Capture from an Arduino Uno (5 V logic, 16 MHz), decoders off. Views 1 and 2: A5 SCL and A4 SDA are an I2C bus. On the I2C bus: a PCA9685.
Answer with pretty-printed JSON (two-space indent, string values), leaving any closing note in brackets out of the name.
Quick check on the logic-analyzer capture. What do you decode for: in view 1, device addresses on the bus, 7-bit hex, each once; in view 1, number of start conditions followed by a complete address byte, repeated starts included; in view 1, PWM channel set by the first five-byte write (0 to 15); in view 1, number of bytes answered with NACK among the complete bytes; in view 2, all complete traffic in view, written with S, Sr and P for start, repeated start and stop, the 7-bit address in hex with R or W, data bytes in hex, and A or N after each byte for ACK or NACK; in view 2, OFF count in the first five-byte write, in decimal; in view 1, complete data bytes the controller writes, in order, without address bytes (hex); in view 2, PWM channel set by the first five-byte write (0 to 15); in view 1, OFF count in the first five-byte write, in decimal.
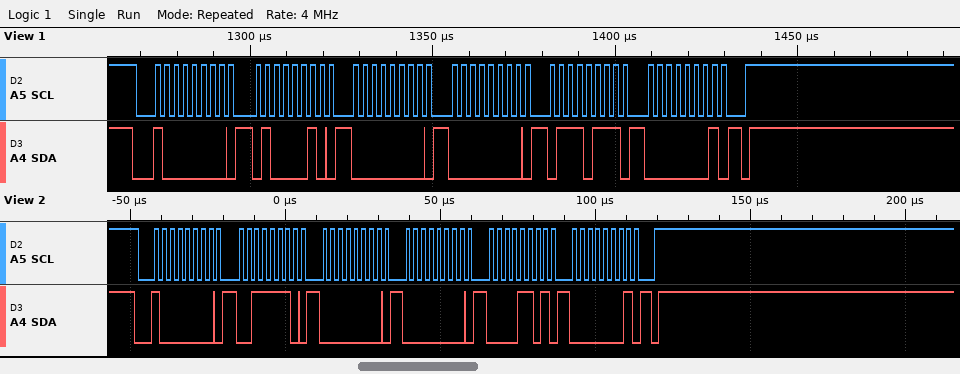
{
  "in view 1, device addresses on the bus, 7-bit hex, each once": "0x40",
  "in view 1, number of start conditions followed by a complete address byte, repeated starts included": "1",
  "in view 1, PWM channel set by the first five-byte write": "15",
  "in view 1, number of bytes answered with NACK among the complete bytes": "0",
  "in view 2, all complete traffic in view, written with S, Sr and P for start, repeated start and stop, the 7-bit address in hex with R or W, data bytes in hex, and A or N after each byte for ACK or NACK": "S 40W A 3E A 00 A 00 A 0D A 01 A P",
  "in view 2, OFF count in the first five-byte write, in decimal": "269",
  "in view 1, complete data bytes the controller writes, in order, without address bytes": "42 00 00 77 01",
  "in view 2, PWM channel set by the first five-byte write": "14",
  "in view 1, OFF count in the first five-byte write, in decimal": "375"
}
